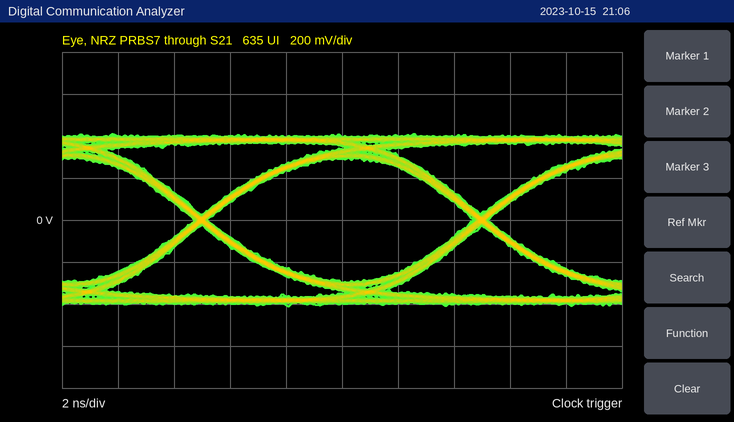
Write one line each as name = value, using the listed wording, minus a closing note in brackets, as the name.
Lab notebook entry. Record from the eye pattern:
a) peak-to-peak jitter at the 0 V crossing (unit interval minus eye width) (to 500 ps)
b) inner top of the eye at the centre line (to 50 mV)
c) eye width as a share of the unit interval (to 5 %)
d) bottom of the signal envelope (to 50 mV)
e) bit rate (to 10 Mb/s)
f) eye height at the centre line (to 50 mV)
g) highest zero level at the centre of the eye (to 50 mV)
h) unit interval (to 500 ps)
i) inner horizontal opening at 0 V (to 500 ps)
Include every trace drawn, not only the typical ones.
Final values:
peak-to-peak jitter at the 0 V crossing (unit interval minus eye width) = 500 ps
inner top of the eye at the centre line = 300 mV
eye width as a share of the unit interval = 95 %
bottom of the signal envelope = -400 mV
bit rate = 100 Mb/s
eye height at the centre line = 600 mV
highest zero level at the centre of the eye = -300 mV
unit interval = 10.0 ns
inner horizontal opening at 0 V = 9.5 ns
